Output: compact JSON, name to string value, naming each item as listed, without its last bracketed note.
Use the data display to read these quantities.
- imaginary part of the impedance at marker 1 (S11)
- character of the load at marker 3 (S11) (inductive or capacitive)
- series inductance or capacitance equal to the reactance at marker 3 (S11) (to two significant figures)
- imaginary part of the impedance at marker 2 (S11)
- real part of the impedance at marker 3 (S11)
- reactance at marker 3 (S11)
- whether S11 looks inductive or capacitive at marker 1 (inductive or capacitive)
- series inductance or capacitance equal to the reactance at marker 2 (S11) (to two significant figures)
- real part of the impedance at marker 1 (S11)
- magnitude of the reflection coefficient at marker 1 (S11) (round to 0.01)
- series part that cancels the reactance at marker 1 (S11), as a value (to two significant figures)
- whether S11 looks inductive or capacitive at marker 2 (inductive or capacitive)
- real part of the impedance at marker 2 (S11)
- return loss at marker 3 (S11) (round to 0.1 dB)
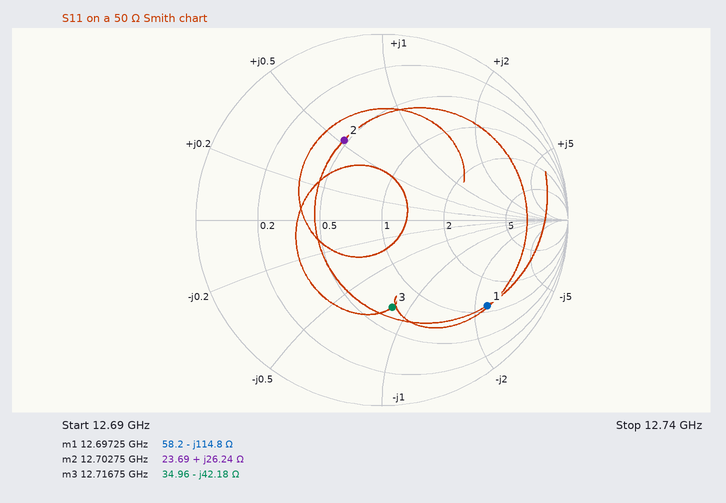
{"imaginary part of the impedance at marker 1": "-114.8 Ω", "character of the load at marker 3 (S11)": "capacitive", "series inductance or capacitance equal to the reactance at marker 3 (S11)": "300 fF", "imaginary part of the impedance at marker 2": "+26.24 Ω", "real part of the impedance at marker 3": "34.96 Ω", "reactance at marker 3": "-42.18 Ω", "whether S11 looks inductive or capacitive at marker 1": "capacitive", "series inductance or capacitance equal to the reactance at marker 2 (S11)": "330 pH", "real part of the impedance at marker 1": "58.2 Ω", "magnitude of the reflection coefficient at marker 1 (S11)": "0.73", "series part that cancels the reactance at marker 1 (S11), as a value": "1.4 nH", "whether S11 looks inductive or capacitive at marker 2": "inductive", "real part of the impedance at marker 2": "23.69 Ω", "return loss at marker 3 (S11)": "6.5 dB"}
